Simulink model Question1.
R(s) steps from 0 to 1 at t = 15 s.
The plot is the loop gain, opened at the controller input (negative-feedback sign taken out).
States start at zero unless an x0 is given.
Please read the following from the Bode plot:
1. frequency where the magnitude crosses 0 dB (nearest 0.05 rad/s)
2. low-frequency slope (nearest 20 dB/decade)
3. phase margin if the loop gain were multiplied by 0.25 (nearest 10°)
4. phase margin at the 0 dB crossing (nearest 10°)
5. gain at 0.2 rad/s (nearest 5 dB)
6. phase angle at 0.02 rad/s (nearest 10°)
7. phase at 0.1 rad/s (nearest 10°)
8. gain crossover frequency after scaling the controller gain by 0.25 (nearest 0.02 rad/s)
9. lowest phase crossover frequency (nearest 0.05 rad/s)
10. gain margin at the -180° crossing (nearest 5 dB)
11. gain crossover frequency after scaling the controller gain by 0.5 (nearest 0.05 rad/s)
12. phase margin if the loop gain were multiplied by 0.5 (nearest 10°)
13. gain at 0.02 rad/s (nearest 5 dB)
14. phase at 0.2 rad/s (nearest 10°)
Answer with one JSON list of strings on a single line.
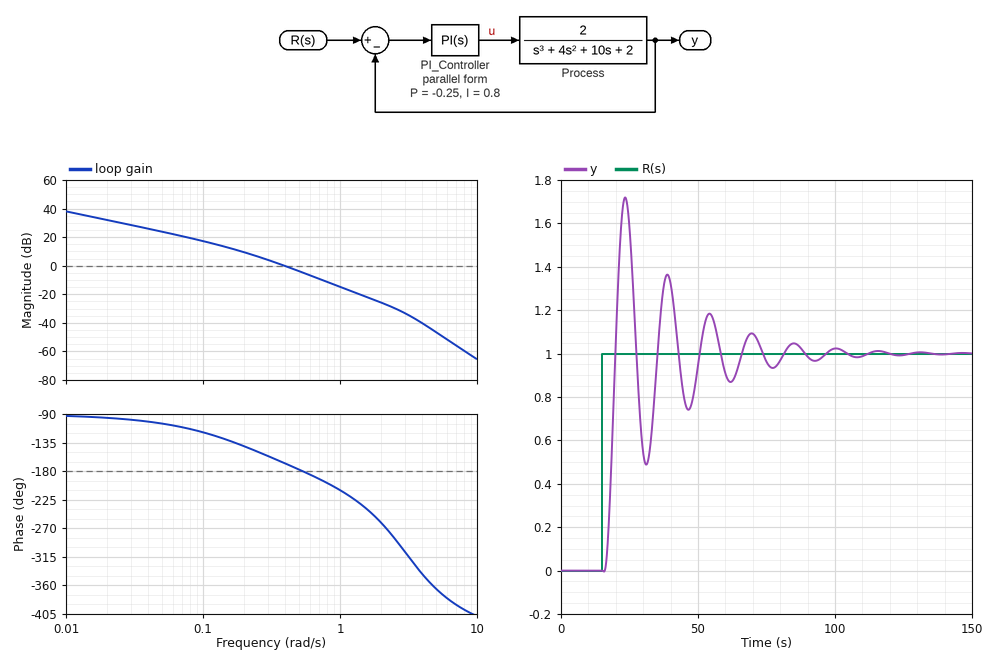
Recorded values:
["0.40 rad/s", "-20 dB/decade", "50°", "10°", "10 dB", "-100°", "-120°", "0.16 rad/s", "0.55 rad/s", "5 dB", "0.25 rad/s", "30°", "30 dB", "-140°"]
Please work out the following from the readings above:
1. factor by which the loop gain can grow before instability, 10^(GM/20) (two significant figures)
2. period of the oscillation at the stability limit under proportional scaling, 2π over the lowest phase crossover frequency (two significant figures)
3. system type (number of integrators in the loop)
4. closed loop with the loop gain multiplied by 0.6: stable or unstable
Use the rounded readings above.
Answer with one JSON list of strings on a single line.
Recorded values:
["1.8", "11 s", "1", "stable"]
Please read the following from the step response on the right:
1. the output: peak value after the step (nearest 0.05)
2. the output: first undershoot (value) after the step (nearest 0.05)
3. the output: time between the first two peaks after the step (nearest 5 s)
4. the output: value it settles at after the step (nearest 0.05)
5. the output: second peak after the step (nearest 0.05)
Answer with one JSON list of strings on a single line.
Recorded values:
["1.70", "0.50", "15 s", "1.00", "1.35"]
